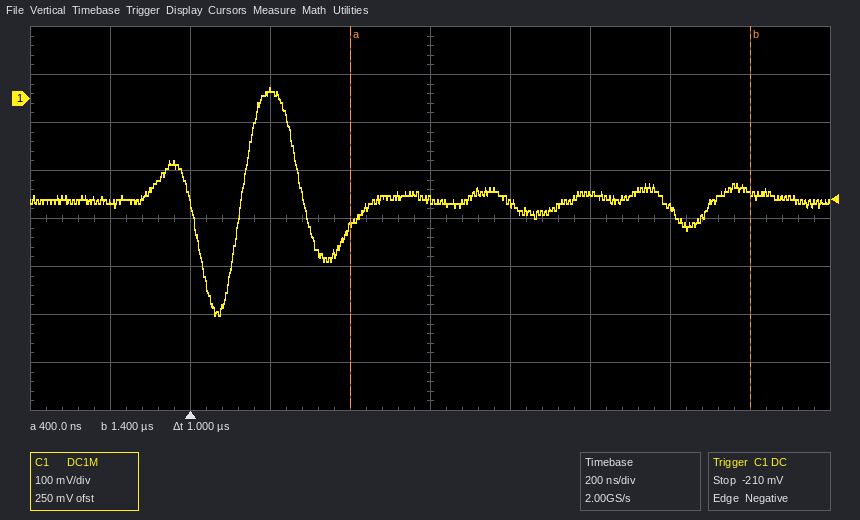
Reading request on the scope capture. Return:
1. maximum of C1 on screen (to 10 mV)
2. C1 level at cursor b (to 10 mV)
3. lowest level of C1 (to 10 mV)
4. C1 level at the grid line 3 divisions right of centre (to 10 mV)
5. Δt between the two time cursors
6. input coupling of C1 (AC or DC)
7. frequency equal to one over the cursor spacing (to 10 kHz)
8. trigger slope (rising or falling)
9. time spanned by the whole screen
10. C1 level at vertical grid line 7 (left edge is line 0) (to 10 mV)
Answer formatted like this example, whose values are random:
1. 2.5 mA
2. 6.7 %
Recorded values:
1. 20 mV
2. -200 mV
3. -450 mV
4. -230 mV
5. 1 µs
6. DC
7. 1.00 MHz
8. falling
9. 2 µs
10. -200 mV
